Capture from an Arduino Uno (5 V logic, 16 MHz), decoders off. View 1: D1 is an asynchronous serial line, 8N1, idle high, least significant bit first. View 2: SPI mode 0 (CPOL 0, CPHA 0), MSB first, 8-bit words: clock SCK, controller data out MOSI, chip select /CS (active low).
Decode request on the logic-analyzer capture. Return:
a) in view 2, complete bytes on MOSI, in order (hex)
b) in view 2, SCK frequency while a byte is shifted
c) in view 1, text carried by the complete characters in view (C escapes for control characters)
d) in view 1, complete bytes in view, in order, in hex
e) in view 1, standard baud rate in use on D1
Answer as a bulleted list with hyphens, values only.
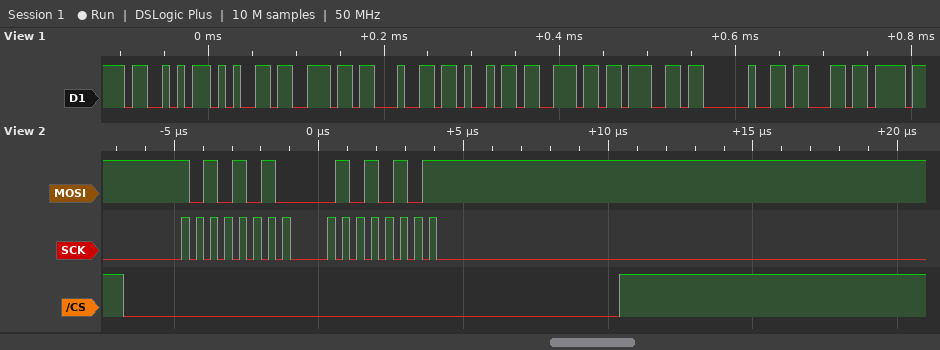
- 0xAA 0x55
- 2 MHz
- "Sending c"
- 0x53 0x65 0x6E 0x64 0x69 0x6E 0x67 0x20 0x63
- 115200 baud
